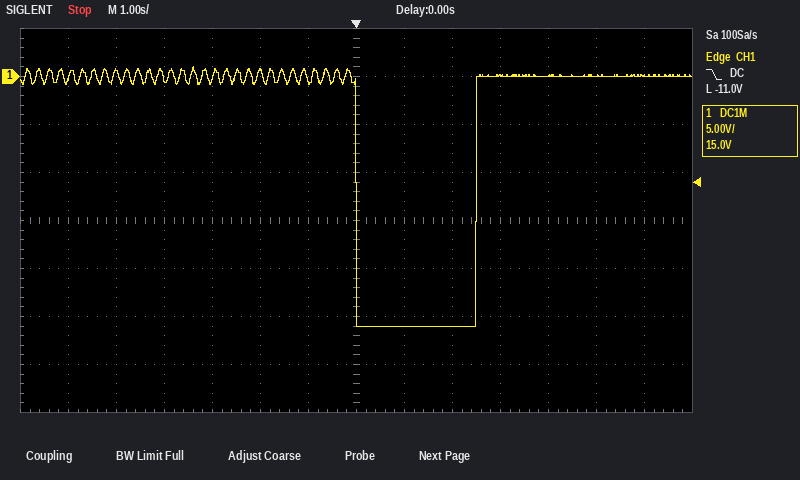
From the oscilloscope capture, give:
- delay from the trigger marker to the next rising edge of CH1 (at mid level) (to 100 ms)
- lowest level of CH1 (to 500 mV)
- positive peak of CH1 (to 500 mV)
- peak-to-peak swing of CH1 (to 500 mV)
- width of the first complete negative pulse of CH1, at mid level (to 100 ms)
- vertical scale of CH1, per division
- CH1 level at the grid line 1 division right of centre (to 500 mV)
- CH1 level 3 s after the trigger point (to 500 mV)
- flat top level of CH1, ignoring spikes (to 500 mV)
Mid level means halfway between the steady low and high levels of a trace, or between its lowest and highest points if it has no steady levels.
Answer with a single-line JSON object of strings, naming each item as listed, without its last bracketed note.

{"delay from the trigger marker to the next rising edge of CH1 (at mid level)": "2.5 s", "lowest level of CH1": "-26.0 V", "positive peak of CH1": "1.0 V", "peak-to-peak swing of CH1": "27.0 V", "width of the first complete negative pulse of CH1, at mid level": "2.5 s", "vertical scale of CH1, per division": "5 V", "CH1 level at the grid line 1 division right of centre": "-26.0 V", "CH1 level 3 s after the trigger point": "0.0 V", "flat top level of CH1, ignoring spikes": "0.0 V"}
